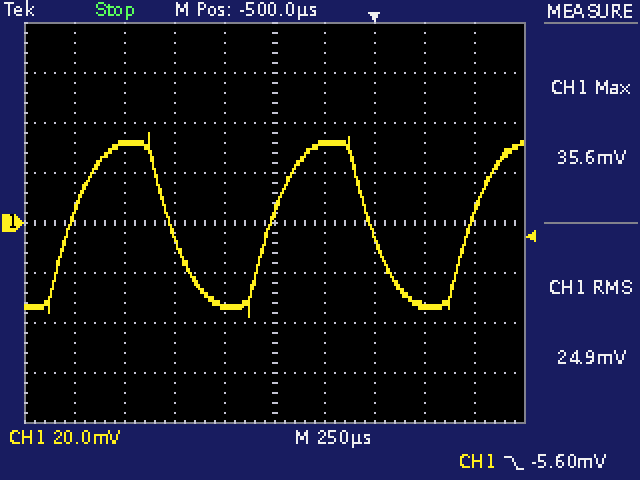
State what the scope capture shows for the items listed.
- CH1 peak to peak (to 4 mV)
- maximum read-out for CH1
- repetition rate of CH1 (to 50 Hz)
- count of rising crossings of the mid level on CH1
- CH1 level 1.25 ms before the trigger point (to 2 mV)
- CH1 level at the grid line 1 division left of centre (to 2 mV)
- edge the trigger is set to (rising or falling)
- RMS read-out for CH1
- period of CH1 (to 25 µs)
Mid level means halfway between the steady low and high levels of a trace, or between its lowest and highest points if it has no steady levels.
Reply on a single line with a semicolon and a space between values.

72 mV; 35.6 mV; 1.00 kHz; 3; 32 mV; -34 mV; falling; 24.9 mV; 1.000 ms
